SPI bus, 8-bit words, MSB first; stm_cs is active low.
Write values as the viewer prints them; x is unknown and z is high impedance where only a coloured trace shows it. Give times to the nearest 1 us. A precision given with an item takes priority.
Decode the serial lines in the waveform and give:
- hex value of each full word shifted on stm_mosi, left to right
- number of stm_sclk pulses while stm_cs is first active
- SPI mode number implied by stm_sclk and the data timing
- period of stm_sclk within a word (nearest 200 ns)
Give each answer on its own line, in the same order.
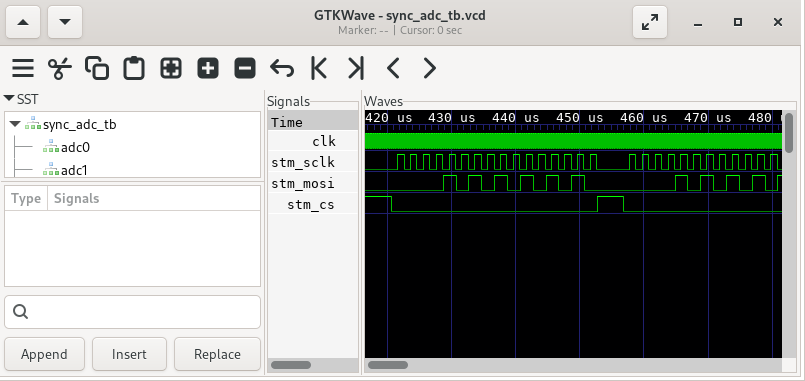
0A, AA, 0A
16
0
2000 ns
